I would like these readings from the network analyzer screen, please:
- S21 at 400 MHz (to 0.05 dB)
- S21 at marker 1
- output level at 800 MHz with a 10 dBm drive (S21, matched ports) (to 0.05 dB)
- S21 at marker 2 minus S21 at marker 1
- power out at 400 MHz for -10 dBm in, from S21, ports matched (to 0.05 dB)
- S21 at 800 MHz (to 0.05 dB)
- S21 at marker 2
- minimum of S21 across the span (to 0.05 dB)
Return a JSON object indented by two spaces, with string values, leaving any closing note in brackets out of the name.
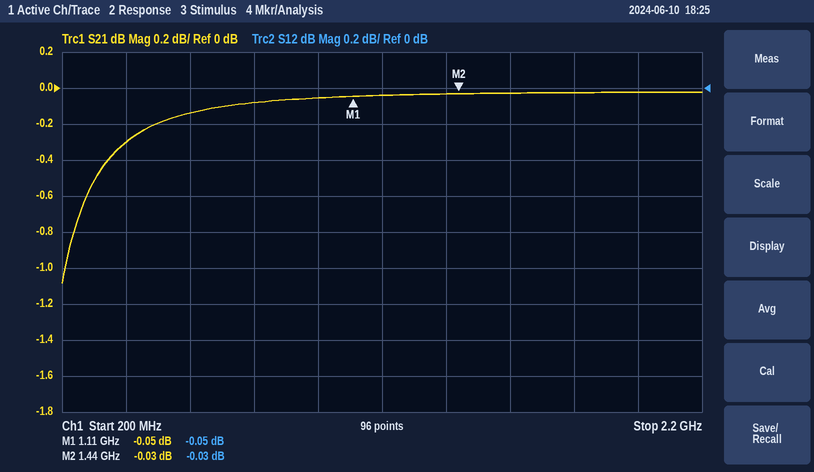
{
  "S21 at 400 MHz": "-0.30 dB",
  "S21 at marker 1": "-0.05 dB",
  "output level at 800 MHz with a 10 dBm drive (S21, matched ports)": "9.90 dBm",
  "S21 at marker 2 minus S21 at marker 1": "0.02 dB",
  "power out at 400 MHz for -10 dBm in, from S21, ports matched": "-10.30 dBm",
  "S21 at 800 MHz": "-0.10 dB",
  "S21 at marker 2": "-0.03 dB",
  "minimum of S21 across the span": "-1.10 dB"
}
